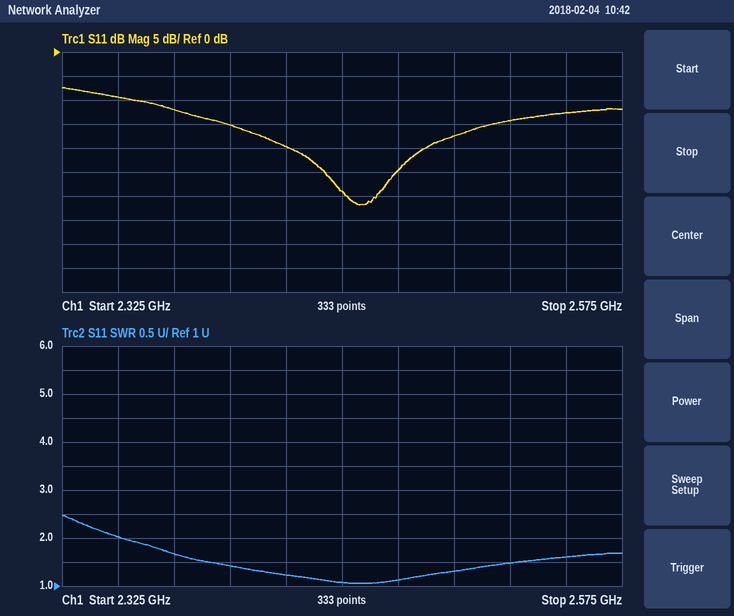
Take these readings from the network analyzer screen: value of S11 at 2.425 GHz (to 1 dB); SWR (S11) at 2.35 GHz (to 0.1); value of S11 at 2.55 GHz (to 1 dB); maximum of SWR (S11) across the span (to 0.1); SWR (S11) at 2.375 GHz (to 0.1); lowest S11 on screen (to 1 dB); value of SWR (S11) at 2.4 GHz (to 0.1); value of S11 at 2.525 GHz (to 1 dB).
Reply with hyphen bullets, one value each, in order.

- -20 dB
- 2.0
- -13 dB
- 2.5
- 1.7
- -32 dB
- 1.4
- -14 dB
